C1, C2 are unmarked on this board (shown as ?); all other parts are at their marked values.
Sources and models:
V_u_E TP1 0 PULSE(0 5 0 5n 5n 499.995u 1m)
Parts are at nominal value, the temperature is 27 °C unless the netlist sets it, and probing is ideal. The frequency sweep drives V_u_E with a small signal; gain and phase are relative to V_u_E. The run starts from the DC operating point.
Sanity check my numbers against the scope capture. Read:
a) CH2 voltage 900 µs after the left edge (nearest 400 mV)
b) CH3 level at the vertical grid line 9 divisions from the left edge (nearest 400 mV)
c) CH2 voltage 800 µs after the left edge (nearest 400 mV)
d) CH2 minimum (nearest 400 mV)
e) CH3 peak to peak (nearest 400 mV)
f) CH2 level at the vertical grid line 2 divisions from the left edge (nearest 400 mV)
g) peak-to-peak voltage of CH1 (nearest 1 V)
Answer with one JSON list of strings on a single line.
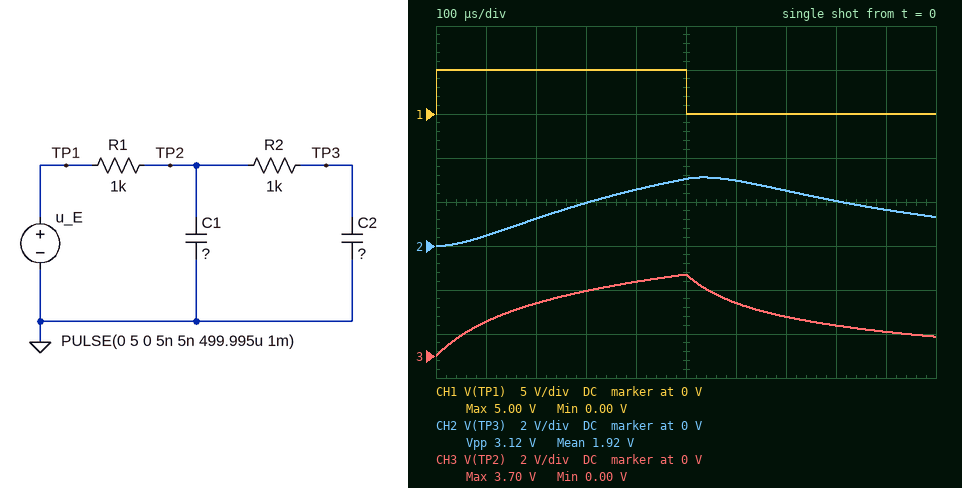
["1.6 V", "1.2 V", "2.0 V", "0 V", "3.6 V", "1.2 V", "5 V"]
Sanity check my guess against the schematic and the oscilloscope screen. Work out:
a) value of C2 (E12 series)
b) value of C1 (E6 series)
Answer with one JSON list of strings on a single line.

["150 nF", "220 nF"]
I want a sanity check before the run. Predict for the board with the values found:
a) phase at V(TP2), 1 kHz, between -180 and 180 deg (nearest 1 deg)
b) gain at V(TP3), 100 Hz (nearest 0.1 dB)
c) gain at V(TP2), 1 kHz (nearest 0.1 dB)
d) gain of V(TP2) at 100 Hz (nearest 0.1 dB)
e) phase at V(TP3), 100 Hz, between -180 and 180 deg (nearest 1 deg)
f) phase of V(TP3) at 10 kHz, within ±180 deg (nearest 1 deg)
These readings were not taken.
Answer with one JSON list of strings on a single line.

["-52 deg", "-0.3 dB", "-7.6 dB", "-0.3 dB", "-18 deg", "-166 deg"]
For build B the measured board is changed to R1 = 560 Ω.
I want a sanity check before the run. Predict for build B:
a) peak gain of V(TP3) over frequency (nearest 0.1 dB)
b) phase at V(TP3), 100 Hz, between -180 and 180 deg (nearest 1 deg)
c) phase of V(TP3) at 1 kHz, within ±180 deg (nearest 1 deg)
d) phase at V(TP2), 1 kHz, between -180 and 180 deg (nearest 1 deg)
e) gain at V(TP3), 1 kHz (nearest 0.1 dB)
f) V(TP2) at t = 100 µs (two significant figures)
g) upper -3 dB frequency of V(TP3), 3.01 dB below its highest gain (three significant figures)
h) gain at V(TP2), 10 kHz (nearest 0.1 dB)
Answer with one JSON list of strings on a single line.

["0 dB", "-13 deg", "-83 deg", "-40 deg", "-7.1 dB", "2.4 V", "518 Hz", "-18.0 dB"]
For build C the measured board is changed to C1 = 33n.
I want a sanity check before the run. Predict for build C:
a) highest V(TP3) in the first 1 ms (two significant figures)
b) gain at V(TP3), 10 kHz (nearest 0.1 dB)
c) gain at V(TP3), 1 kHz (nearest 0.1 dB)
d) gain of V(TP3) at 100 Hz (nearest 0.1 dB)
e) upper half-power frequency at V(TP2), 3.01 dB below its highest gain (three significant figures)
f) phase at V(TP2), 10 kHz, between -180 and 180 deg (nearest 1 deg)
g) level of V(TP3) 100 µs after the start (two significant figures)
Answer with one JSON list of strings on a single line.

["3.9 V", "-28.9 dB", "-7.0 dB", "-0.2 dB", "670 Hz", "-48 deg", "1.2 V"]
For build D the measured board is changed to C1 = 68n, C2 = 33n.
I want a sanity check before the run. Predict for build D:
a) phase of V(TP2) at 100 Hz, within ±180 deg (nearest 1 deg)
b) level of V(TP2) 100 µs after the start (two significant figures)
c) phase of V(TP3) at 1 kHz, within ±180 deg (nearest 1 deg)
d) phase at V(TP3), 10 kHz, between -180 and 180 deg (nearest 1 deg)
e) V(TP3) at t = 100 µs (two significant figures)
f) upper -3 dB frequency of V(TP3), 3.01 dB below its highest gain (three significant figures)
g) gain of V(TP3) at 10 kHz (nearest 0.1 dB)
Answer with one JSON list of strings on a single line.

["-4 deg", "3.2 V", "-43 deg", "-133 deg", "2.5 V", "1.35 kHz", "-21.2 dB"]
